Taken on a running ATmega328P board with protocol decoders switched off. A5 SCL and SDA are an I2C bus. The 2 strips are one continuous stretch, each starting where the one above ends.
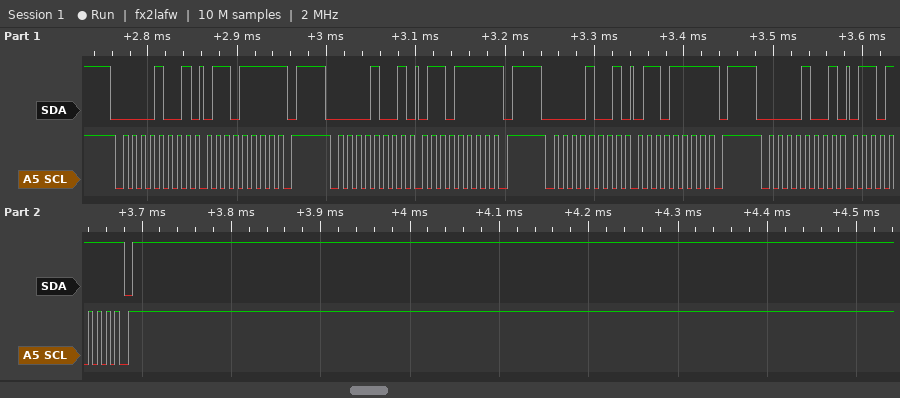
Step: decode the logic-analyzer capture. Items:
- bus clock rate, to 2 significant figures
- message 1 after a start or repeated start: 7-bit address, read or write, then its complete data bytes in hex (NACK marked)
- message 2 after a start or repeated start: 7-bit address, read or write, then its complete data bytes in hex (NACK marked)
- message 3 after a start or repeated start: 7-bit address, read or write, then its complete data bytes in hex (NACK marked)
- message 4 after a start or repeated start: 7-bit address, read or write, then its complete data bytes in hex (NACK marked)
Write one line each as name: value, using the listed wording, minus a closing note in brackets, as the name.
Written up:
bus clock rate, to 2 significant figures: 100 kHz
message 1 after a start or repeated start: 7-bit address, read or write, then its complete data bytes in hex: 0x04 read: 6F NACK
message 2 after a start or repeated start: 7-bit address, read or write, then its complete data bytes in hex: 0x04 read: 6F NACK
message 3 after a start or repeated start: 7-bit address, read or write, then its complete data bytes in hex: 0x04 read: 6F NACK
message 4 after a start or repeated start: 7-bit address, read or write, then its complete data bytes in hex: 0x04 read: 6F NACK
